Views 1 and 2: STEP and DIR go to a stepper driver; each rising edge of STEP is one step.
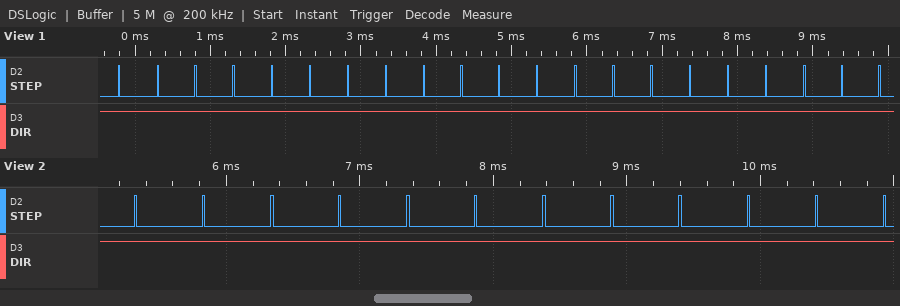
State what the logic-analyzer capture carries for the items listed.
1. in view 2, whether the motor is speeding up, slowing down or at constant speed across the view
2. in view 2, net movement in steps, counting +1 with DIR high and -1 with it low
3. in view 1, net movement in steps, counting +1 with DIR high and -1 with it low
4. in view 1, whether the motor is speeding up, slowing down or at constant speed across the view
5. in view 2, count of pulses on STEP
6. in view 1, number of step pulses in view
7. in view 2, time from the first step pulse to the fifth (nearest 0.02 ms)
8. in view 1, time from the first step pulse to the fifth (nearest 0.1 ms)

constant speed
+12
+21
constant speed
12
21
2.04 ms
2.0 ms
